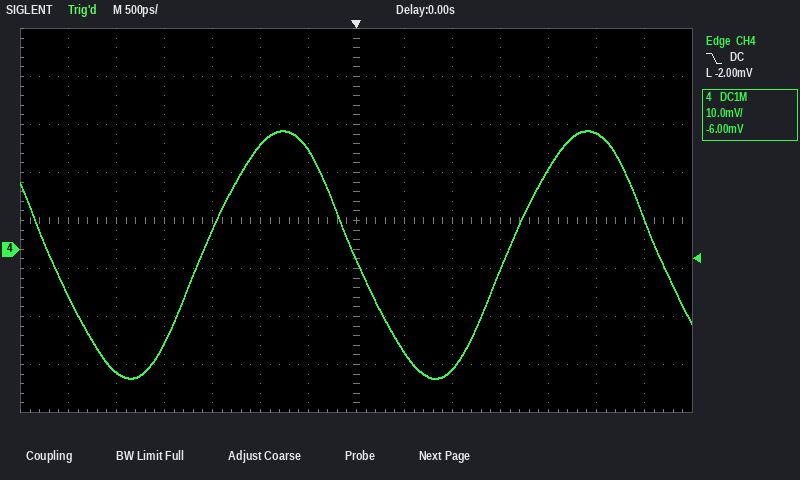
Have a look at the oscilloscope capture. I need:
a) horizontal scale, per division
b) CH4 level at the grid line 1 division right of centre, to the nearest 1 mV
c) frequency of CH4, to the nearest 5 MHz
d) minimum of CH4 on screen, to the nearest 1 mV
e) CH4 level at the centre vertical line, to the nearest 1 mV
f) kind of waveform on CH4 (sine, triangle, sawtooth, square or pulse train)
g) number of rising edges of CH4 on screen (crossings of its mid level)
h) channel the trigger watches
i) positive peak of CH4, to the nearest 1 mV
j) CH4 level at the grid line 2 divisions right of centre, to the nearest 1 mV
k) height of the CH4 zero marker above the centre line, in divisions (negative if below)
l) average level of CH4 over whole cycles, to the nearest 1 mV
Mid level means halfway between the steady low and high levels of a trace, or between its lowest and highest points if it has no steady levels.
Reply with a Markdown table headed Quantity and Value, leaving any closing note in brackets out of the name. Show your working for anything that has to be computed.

| Quantity | Value |
|---|---|
| horizontal scale, per division | 500 ps |
| CH4 level at the grid line 1 division right of centre, to the nearest 1 mV | -21 mV |
| frequency of CH4, to the nearest 5 MHz | 315 MHz |
| minimum of CH4 on screen, to the nearest 1 mV | -27 mV |
| CH4 level at the centre vertical line, to the nearest 1 mV | -2 mV |
| kind of waveform on CH4 | sine |
| number of rising edges of CH4 on screen | 2 |
| channel the trigger watches | CH4 |
| positive peak of CH4, to the nearest 1 mV | 25 mV |
| CH4 level at the grid line 2 divisions right of centre, to the nearest 1 mV | -25 mV |
| height of the CH4 zero marker above the centre line, in divisions | -0.6 div |
| average level of CH4 over whole cycles, to the nearest 1 mV | (25 mV + (-27 mV)) / 2 ≈ -1 mV |
